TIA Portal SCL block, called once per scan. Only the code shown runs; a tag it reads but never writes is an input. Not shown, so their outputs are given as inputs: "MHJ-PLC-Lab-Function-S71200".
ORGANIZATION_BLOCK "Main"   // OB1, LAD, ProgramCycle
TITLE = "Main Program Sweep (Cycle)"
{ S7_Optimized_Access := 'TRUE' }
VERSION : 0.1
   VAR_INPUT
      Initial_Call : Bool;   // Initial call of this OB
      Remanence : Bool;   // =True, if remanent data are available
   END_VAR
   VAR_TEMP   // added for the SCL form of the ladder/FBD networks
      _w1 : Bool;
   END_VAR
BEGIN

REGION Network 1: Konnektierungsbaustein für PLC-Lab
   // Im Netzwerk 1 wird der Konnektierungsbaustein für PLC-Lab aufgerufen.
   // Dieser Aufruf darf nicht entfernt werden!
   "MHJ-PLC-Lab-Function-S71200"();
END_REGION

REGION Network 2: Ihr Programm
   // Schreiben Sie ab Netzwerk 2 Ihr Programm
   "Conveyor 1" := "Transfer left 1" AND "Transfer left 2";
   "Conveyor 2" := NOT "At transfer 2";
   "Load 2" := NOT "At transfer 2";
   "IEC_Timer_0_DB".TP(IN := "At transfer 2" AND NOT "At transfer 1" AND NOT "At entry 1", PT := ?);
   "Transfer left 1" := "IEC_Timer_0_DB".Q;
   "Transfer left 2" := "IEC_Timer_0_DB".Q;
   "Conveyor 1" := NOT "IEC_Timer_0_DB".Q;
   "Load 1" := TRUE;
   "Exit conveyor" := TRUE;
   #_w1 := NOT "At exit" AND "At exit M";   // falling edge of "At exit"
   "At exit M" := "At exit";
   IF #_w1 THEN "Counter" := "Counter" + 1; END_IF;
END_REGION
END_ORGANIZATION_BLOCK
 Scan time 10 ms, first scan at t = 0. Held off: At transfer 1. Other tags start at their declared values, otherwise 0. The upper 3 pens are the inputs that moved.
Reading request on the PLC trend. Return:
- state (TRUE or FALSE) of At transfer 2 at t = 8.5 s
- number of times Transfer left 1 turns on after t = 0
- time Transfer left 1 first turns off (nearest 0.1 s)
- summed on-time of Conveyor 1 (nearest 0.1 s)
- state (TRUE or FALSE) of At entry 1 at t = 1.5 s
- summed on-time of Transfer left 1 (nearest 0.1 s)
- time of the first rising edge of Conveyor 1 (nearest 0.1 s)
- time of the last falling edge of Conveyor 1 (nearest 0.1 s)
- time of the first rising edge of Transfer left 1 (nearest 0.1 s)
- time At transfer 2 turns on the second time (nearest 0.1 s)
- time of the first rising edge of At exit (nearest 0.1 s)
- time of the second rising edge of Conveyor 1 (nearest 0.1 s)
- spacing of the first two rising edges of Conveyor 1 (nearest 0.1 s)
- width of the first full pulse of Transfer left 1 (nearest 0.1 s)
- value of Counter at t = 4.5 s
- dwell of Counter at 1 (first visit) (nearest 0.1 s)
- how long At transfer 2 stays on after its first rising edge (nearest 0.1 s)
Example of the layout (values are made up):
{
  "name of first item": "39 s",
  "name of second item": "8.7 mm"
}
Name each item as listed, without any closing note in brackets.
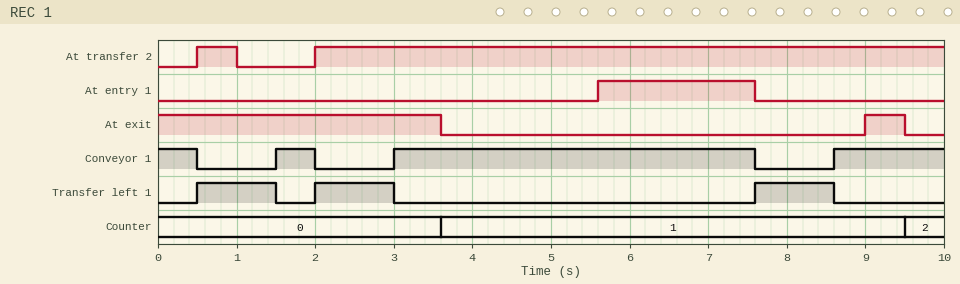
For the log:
{
  "state (TRUE or FALSE) of At transfer 2 at t = 8.5 s": "TRUE",
  "number of times Transfer left 1 turns on after t = 0": "3",
  "time Transfer left 1 first turns off": "1.5 s",
  "summed on-time of Conveyor 1": "7.0 s",
  "state (TRUE or FALSE) of At entry 1 at t = 1.5 s": "FALSE",
  "summed on-time of Transfer left 1": "3.0 s",
  "time of the first rising edge of Conveyor 1": "1.5 s",
  "time of the last falling edge of Conveyor 1": "7.6 s",
  "time of the first rising edge of Transfer left 1": "0.5 s",
  "time At transfer 2 turns on the second time": "2.0 s",
  "time of the first rising edge of At exit": "9.0 s",
  "time of the second rising edge of Conveyor 1": "3.0 s",
  "spacing of the first two rising edges of Conveyor 1": "1.5 s",
  "width of the first full pulse of Transfer left 1": "1.0 s",
  "value of Counter at t = 4.5 s": "1",
  "dwell of Counter at 1 (first visit)": "5.9 s",
  "how long At transfer 2 stays on after its first rising edge": "0.5 s"
}
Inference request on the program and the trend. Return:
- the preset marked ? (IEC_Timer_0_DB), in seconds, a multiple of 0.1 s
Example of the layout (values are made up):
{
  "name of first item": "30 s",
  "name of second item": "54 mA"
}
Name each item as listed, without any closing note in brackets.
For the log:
{
  "the preset marked ? (IEC_Timer_0_DB), in seconds, a multiple of 0.1 s": "1.0 s"
}
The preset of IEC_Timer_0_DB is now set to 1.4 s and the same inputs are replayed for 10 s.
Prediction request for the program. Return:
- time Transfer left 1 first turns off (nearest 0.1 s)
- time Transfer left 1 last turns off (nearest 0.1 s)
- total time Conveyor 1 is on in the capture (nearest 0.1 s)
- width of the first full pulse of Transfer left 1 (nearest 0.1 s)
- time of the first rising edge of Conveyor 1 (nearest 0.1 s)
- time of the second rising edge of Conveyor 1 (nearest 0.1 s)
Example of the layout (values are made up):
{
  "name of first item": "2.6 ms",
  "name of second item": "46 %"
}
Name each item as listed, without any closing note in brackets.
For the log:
{
  "time Transfer left 1 first turns off": "1.9 s",
  "time Transfer left 1 last turns off": "9.0 s",
  "total time Conveyor 1 is on in the capture": "5.8 s",
  "width of the first full pulse of Transfer left 1": "1.4 s",
  "time of the first rising edge of Conveyor 1": "1.9 s",
  "time of the second rising edge of Conveyor 1": "3.4 s"
}
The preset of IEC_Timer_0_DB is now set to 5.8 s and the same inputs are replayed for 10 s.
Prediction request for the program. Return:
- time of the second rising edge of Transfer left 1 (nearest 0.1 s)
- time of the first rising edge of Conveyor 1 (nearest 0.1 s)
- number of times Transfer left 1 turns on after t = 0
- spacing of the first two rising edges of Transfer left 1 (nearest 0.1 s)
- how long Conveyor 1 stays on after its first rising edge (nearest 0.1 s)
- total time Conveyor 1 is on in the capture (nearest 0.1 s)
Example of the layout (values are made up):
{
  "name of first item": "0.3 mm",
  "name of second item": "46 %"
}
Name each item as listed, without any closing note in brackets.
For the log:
{
  "time of the second rising edge of Transfer left 1": "7.6 s",
  "time of the first rising edge of Conveyor 1": "6.3 s",
  "number of times Transfer left 1 turns on after t = 0": "2",
  "spacing of the first two rising edges of Transfer left 1": "7.1 s",
  "how long Conveyor 1 stays on after its first rising edge": "1.3 s",
  "total time Conveyor 1 is on in the capture": "1.8 s"
}
